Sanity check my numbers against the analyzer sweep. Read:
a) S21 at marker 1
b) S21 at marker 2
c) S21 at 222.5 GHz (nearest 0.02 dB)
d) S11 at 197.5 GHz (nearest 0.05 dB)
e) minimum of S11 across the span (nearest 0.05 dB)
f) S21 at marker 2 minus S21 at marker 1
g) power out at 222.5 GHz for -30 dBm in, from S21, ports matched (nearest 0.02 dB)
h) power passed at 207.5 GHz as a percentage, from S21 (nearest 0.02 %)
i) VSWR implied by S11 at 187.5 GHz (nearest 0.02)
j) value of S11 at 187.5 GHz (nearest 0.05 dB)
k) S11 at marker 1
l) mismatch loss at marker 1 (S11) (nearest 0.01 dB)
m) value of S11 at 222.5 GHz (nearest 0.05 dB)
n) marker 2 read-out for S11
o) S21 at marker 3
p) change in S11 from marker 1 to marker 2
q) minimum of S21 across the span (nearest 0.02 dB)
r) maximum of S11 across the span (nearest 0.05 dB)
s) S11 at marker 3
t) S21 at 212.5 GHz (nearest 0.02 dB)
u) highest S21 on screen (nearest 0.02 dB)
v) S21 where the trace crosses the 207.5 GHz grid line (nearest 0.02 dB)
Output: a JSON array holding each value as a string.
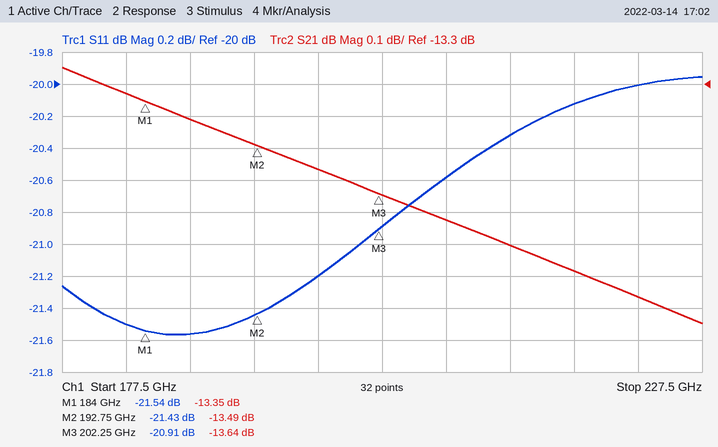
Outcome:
["-13.35 dB", "-13.49 dB", "-13.96 dB", "-21.20 dB", "-21.55 dB", "-0.14 dB", "-43.96 dBm", "4.24 %", "1.18", "-21.55 dB", "-21.54 dB", "0.03 dB", "-20.00 dB", "-21.43 dB", "-13.64 dB", "0.11 dB", "-14.04 dB", "-19.95 dB", "-20.91 dB", "-13.80 dB", "-13.24 dB", "-13.72 dB"]
